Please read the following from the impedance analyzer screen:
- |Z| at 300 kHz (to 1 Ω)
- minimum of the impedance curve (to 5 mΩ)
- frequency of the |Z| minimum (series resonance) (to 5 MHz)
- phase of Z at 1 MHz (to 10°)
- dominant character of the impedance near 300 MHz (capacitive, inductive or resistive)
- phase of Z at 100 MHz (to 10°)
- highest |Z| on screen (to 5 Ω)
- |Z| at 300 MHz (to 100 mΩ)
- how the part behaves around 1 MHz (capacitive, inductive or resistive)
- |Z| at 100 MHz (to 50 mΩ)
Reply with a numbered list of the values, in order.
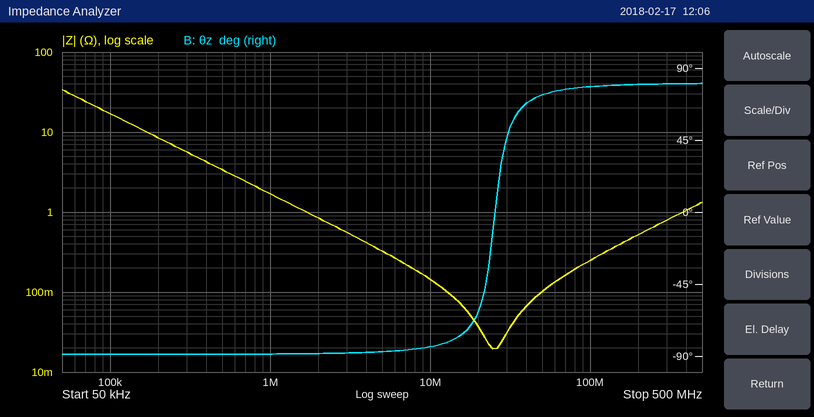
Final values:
1. 6 Ω
2. 20 mΩ
3. 25 MHz
4. -90°
5. inductive
6. 80°
7. 35 Ω
8. 800 mΩ
9. capacitive
10. 250 mΩ
